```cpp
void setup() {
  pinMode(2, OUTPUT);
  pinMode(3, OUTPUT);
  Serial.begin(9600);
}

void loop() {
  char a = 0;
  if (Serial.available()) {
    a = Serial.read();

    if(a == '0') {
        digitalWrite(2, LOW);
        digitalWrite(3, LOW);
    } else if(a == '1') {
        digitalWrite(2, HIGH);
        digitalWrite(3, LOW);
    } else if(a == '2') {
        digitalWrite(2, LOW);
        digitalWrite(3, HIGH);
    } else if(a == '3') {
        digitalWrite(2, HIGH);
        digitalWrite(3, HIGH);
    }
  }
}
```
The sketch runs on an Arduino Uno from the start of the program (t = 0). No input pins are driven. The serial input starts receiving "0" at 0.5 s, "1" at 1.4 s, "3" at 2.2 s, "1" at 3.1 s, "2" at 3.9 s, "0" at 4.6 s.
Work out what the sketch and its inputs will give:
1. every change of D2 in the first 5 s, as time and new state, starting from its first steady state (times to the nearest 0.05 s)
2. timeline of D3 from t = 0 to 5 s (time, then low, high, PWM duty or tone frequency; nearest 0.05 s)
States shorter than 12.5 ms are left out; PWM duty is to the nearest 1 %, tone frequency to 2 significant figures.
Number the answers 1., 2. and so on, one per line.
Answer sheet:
1. 0 s low; 1.4 s high; 3.9 s low
2. 0 s low; 2.2 s high; 3.1 s low; 3.9 s high; 4.6 s low
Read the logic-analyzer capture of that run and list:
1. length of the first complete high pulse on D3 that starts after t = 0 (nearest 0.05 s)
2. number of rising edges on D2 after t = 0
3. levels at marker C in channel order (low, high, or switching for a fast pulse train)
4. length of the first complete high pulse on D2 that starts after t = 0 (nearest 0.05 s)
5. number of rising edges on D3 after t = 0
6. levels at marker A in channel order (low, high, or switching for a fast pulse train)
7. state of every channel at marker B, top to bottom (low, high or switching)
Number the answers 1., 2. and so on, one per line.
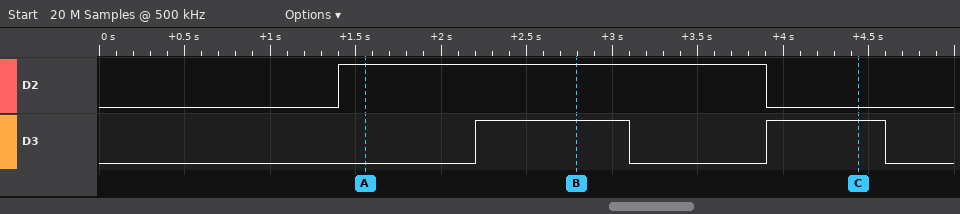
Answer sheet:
1. 0.90 s
2. 1
3. D2 low, D3 high
4. 2.50 s
5. 2
6. D2 high, D3 low
7. D2 high, D3 high
